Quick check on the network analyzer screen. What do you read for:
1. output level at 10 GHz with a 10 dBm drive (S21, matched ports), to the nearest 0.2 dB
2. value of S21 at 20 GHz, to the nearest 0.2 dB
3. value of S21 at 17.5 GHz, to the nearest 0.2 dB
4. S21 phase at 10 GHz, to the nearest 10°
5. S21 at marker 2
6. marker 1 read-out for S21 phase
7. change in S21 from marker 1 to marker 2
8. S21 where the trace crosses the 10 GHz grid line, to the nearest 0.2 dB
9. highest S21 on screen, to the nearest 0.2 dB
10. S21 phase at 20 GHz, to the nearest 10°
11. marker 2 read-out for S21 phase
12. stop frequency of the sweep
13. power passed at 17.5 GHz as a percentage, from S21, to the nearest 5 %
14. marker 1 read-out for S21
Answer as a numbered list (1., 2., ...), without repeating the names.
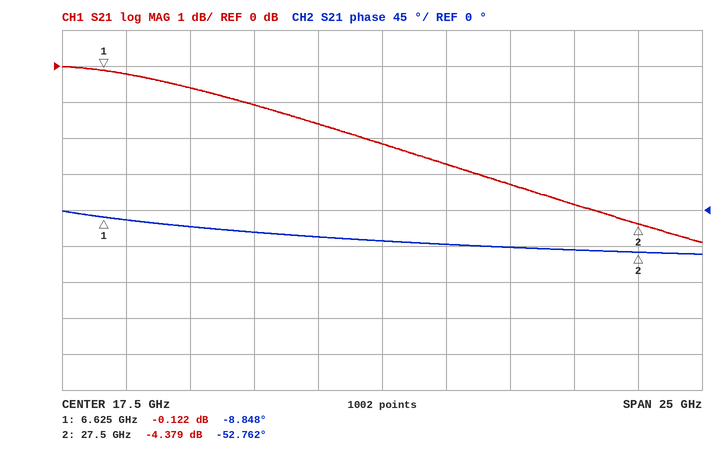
1. 9.4 dBm
2. -2.8 dB
3. -2.2 dB
4. -20°
5. -4.379 dB
6. -8.848°
7. -4.257 dB
8. -0.6 dB
9. 0.0 dB
10. -40°
11. -52.762°
12. 30 GHz
13. 60 %
14. -0.122 dB
